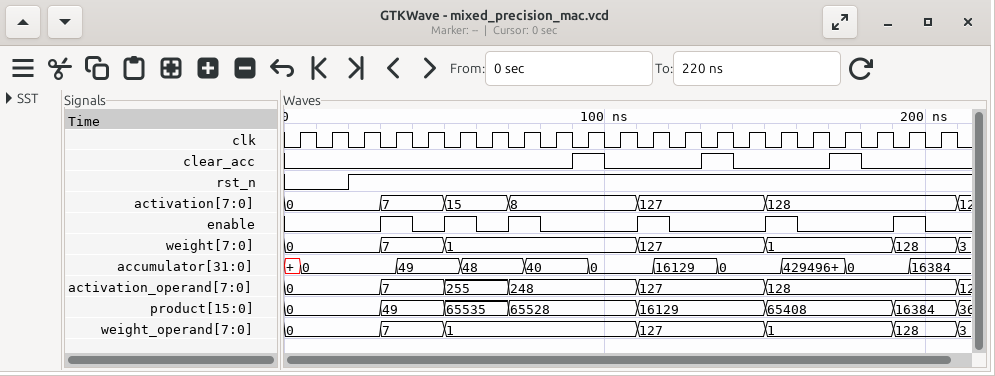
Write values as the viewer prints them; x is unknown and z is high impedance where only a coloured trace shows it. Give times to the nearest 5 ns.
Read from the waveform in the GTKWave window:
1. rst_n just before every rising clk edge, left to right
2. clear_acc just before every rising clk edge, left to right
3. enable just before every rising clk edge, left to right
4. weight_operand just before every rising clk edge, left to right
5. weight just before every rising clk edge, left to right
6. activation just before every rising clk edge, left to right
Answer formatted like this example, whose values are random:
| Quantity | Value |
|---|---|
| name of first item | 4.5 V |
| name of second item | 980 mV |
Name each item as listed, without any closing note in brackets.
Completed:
| Quantity | Value |
|---|---|
| rst_n just before every rising clk edge, left to right | 0 0 1 1 1 1 1 1 1 1 1 1 1 1 1 1 1 1 1 1 1 |
| clear_acc just before every rising clk edge, left to right | 0 0 0 0 0 0 0 0 0 1 0 0 0 1 0 0 0 1 0 0 0 |
| enable just before every rising clk edge, left to right | 0 0 0 1 0 1 0 1 0 0 0 1 0 0 0 1 0 0 0 1 0 |
| weight_operand just before every rising clk edge, left to right | 0, 0, 0, 7, 7, 1, 1, 1, 1, 1, 1, 127, 127, 127, 127, 1, 1, 1, 1, 128, 128 |
| weight just before every rising clk edge, left to right | 0, 0, 0, 7, 7, 1, 1, 1, 1, 1, 1, 127, 127, 127, 127, 1, 1, 1, 1, 128, 128 |
| activation just before every rising clk edge, left to right | 0, 0, 0, 7, 7, 15, 15, 8, 8, 8, 8, 127, 127, 127, 127, 128, 128, 128, 128, 128, 128 |
